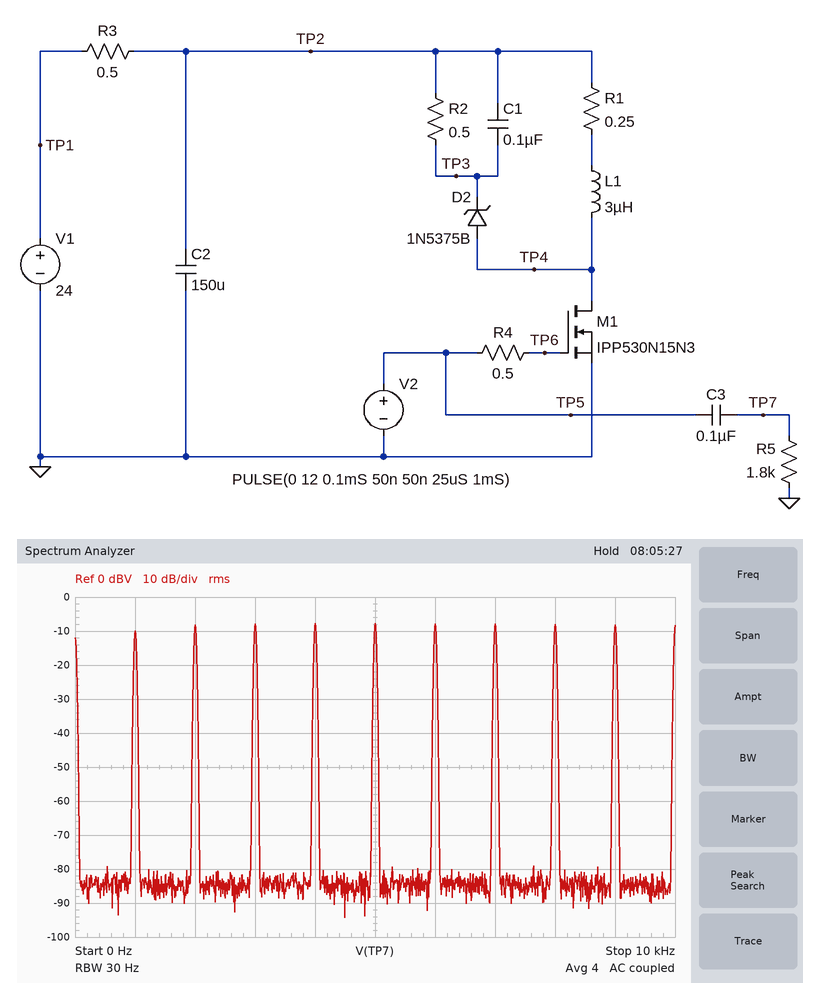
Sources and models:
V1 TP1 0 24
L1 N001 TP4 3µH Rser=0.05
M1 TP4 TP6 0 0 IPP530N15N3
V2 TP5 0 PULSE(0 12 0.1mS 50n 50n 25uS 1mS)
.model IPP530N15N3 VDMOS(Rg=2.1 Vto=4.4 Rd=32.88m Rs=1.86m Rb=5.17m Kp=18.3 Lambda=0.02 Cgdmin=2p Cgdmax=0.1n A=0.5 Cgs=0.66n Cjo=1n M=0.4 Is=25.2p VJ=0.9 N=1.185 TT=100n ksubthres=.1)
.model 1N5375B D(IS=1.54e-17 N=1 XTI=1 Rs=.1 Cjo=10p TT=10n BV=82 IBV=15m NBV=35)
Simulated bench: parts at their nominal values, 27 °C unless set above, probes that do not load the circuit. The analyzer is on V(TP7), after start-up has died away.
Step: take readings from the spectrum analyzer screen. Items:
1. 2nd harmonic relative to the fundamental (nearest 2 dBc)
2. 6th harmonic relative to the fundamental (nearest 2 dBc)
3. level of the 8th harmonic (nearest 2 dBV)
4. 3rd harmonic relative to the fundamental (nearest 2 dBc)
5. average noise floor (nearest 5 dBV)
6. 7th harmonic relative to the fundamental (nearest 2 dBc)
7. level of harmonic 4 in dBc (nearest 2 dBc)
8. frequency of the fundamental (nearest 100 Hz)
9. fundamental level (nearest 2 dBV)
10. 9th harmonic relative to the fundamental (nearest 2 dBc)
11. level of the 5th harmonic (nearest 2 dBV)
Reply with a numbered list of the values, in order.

1. 2 dBc
2. 2 dBc
3. -8 dBV
4. 2 dBc
5. -85 dBV
6. 2 dBc
7. 2 dBc
8. 1.0 kHz
9. -10 dBV
10. 2 dBc
11. -8 dBV
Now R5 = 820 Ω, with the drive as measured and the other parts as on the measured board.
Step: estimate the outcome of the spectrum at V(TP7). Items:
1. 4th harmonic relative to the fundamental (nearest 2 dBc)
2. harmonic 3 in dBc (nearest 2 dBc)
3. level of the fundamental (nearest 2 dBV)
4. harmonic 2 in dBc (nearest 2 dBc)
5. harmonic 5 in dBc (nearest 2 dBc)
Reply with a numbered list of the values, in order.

1. 6 dBc
2. 6 dBc
3. -14 dBV
4. 4 dBc
5. 6 dBc
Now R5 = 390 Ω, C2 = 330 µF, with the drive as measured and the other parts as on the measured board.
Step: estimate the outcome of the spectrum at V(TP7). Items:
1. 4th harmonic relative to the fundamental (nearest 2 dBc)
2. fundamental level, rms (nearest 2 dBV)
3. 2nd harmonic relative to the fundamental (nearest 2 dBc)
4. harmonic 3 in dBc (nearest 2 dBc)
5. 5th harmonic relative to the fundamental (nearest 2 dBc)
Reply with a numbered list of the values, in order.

1. 10 dBc
2. -20 dBV
3. 6 dBc
4. 8 dBc
5. 10 dBc
